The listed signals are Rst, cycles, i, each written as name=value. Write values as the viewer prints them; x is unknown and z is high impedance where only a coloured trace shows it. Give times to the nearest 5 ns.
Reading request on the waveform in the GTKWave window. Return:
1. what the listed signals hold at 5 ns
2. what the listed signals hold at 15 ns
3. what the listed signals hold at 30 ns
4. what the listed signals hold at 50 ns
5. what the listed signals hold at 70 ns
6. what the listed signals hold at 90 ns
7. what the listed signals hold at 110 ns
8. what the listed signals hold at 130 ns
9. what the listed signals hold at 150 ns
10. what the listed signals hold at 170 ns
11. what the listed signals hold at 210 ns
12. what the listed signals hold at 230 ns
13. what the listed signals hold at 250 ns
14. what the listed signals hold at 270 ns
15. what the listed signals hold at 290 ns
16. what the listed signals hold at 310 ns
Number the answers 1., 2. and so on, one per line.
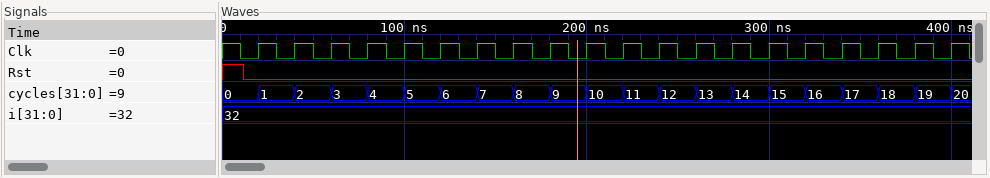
1. Rst=1, cycles=0, i=32
2. Rst=0, cycles=0, i=32
3. Rst=0, cycles=1, i=32
4. Rst=0, cycles=2, i=32
5. Rst=0, cycles=3, i=32
6. Rst=0, cycles=4, i=32
7. Rst=0, cycles=5, i=32
8. Rst=0, cycles=6, i=32
9. Rst=0, cycles=7, i=32
10. Rst=0, cycles=8, i=32
11. Rst=0, cycles=10, i=32
12. Rst=0, cycles=11, i=32
13. Rst=0, cycles=12, i=32
14. Rst=0, cycles=13, i=32
15. Rst=0, cycles=14, i=32
16. Rst=0, cycles=15, i=32
